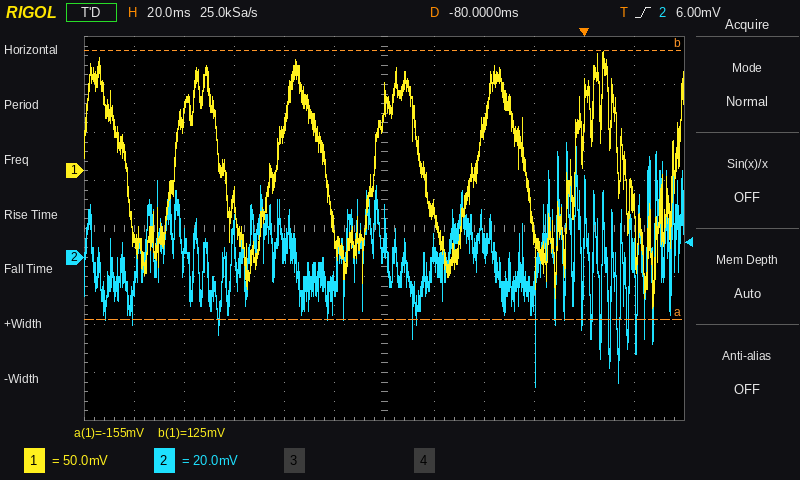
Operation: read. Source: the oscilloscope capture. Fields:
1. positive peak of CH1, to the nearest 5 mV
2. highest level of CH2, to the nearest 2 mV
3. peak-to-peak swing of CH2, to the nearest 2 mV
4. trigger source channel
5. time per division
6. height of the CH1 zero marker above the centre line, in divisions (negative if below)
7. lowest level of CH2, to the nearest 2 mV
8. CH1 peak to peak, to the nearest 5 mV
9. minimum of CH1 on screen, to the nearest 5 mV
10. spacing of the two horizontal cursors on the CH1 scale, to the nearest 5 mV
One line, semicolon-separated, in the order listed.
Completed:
125 mV; 48 mV; 102 mV; CH2; 20 ms; +1.2 div; -54 mV; 265 mV; -140 mV; 280 mV
